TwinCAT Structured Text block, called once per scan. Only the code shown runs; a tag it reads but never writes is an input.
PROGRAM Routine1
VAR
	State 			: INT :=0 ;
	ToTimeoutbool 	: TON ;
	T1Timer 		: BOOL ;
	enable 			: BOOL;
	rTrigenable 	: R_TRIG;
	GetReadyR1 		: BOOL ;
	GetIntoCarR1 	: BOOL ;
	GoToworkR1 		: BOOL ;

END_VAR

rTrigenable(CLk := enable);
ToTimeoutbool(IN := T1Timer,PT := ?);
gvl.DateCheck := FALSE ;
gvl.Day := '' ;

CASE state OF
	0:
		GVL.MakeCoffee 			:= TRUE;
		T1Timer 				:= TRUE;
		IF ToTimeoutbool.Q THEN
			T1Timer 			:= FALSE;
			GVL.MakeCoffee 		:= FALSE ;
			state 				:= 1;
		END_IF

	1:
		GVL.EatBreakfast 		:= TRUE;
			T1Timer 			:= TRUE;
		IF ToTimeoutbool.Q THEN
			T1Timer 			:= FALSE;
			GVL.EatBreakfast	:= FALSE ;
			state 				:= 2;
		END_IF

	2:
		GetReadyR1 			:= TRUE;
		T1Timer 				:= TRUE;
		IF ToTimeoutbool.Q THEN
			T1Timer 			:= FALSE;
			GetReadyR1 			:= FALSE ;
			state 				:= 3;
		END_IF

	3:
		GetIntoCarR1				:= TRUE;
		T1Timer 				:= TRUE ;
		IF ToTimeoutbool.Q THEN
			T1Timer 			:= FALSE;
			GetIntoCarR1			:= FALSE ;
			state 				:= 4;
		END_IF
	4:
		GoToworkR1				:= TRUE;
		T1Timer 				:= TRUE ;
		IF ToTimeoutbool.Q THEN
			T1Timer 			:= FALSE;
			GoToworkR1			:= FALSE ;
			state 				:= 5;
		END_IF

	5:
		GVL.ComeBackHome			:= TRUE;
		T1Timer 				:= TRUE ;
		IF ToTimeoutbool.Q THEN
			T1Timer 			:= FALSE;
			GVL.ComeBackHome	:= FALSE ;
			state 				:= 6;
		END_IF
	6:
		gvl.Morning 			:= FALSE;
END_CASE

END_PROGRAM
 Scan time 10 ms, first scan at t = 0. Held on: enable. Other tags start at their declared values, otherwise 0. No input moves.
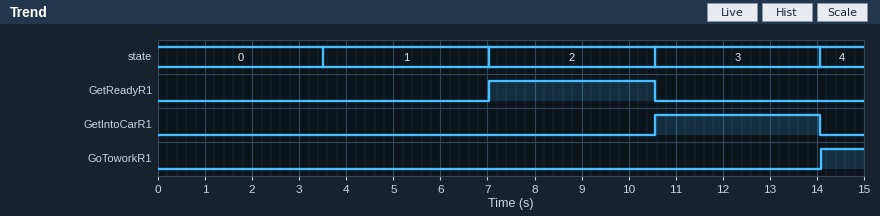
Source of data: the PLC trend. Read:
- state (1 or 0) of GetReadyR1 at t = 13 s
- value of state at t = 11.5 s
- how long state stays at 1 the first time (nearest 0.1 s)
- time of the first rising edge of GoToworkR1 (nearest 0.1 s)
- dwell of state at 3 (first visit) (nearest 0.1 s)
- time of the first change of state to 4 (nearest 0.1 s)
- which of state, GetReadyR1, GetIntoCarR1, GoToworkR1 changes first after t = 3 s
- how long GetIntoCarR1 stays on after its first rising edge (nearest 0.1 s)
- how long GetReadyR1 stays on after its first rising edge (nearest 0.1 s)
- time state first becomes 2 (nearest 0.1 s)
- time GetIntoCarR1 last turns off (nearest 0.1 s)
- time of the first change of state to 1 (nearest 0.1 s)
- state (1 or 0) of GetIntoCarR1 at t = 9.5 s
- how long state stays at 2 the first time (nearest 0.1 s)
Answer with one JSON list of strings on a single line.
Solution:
["0", "3", "3.5 s", "14.1 s", "3.5 s", "14.1 s", "state", "3.5 s", "3.5 s", "7.0 s", "14.1 s", "3.5 s", "0", "3.5 s"]
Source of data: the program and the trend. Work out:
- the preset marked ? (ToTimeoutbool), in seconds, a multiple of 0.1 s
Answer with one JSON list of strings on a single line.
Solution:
["3.5 s"]
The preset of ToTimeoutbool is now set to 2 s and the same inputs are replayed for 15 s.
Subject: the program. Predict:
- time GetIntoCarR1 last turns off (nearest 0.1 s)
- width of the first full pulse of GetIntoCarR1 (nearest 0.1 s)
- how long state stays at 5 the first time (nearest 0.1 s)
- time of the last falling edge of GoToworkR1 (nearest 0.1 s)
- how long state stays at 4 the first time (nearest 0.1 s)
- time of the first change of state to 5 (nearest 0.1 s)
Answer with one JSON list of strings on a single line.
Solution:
["8.1 s", "2.0 s", "2.0 s", "10.1 s", "2.0 s", "10.1 s"]
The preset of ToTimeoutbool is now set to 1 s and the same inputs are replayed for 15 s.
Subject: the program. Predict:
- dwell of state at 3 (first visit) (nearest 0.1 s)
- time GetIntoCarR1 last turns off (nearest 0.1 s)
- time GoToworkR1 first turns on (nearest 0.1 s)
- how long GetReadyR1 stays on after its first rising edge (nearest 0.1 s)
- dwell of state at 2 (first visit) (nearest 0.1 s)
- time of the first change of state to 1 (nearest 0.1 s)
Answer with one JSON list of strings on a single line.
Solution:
["1.0 s", "4.1 s", "4.1 s", "1.0 s", "1.0 s", "1.0 s"]
